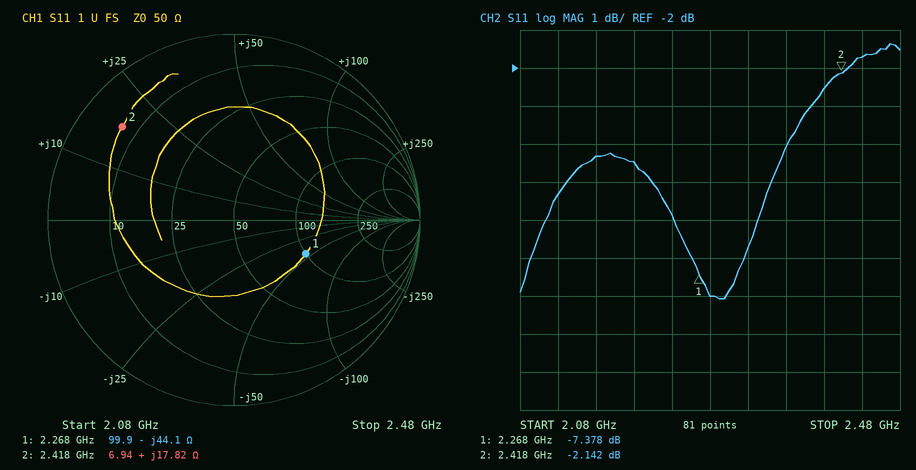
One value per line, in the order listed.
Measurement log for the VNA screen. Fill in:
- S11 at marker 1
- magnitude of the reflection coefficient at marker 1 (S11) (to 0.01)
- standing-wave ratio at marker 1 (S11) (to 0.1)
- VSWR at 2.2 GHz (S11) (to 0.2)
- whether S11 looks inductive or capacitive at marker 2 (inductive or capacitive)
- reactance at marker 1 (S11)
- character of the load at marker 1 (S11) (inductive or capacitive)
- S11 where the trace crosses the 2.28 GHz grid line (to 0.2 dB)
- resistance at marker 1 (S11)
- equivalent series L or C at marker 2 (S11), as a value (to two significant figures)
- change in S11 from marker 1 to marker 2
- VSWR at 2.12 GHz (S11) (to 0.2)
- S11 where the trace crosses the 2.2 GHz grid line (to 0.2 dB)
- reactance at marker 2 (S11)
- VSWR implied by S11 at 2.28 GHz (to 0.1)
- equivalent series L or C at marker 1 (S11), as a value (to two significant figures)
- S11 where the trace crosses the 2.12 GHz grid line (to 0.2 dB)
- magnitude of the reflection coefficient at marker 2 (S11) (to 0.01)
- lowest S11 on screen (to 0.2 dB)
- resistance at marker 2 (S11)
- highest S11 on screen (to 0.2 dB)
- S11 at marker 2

-7.378 dB
0.43
2.5
4.0
inductive
-44.1 Ω
capacitive
-8.0 dB
99.9 Ω
1.2 nH
5.236 dB
3.4
-4.4 dB
+17.82 Ω
2.3
1.6 pF
-5.4 dB
0.78
-8.0 dB
6.94 Ω
-1.4 dB
-2.142 dB
